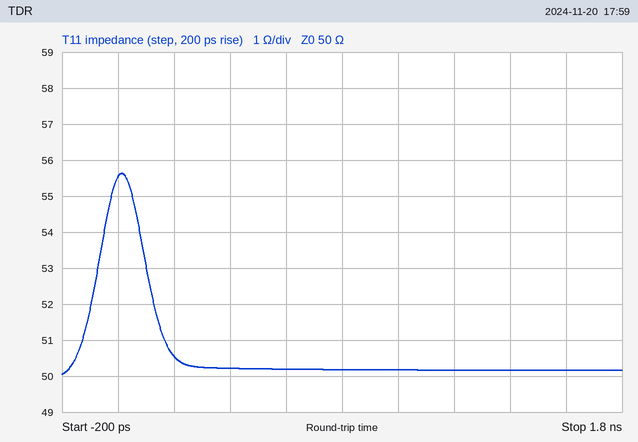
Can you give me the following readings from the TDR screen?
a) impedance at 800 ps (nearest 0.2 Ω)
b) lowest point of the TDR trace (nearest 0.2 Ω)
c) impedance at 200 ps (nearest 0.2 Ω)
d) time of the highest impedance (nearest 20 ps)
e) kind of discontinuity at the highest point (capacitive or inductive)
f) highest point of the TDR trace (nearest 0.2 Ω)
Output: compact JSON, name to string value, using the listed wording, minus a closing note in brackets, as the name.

{"impedance at 800 ps": "50.2 Ω", "lowest point of the TDR trace": "50.0 Ω", "impedance at 200 ps": "50.6 Ω", "time of the highest impedance": "20 ps", "kind of discontinuity at the highest point": "inductive", "highest point of the TDR trace": "55.6 Ω"}
